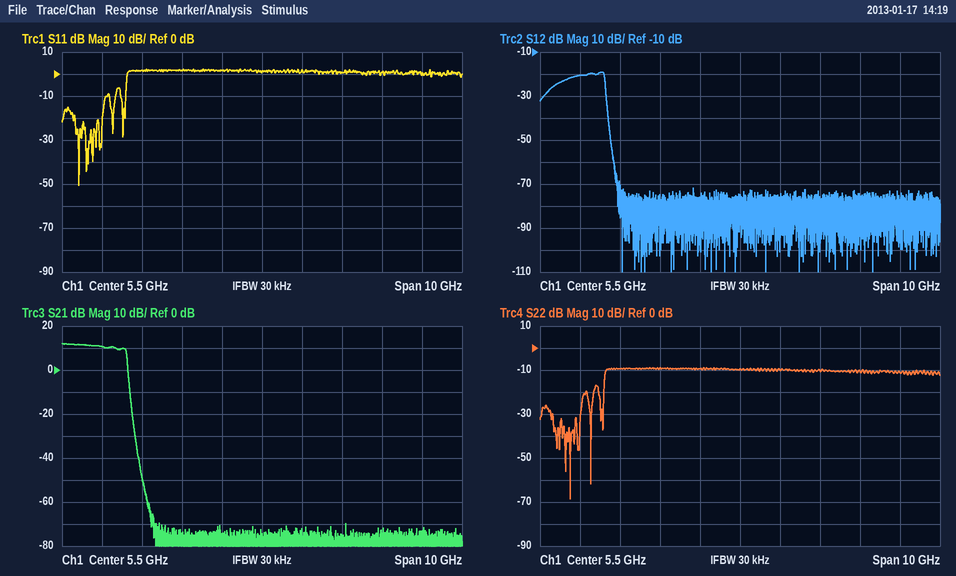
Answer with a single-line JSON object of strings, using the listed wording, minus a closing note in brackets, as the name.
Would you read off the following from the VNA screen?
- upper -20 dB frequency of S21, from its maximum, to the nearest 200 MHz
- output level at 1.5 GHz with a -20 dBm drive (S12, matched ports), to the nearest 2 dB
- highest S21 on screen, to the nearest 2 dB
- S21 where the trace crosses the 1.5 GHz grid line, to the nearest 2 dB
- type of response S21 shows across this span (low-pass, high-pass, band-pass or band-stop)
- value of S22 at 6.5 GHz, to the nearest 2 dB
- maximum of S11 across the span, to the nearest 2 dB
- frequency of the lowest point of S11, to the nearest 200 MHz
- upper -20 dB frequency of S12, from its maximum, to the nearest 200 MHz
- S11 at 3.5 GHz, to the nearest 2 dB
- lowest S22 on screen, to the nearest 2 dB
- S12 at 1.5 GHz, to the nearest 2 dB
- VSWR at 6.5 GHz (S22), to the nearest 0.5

{"upper -20 dB frequency of S21, from its maximum, to the nearest 200 MHz": "2.2 GHz", "output level at 1.5 GHz with a -20 dBm drive (S12, matched ports), to the nearest 2 dB": "-40 dBm", "highest S21 on screen, to the nearest 2 dB": "12 dB", "S21 where the trace crosses the 1.5 GHz grid line, to the nearest 2 dB": "10 dB", "type of response S21 shows across this span": "low-pass", "value of S22 at 6.5 GHz, to the nearest 2 dB": "-10 dB", "maximum of S11 across the span, to the nearest 2 dB": "2 dB", "frequency of the lowest point of S11, to the nearest 200 MHz": "1.0 GHz", "upper -20 dB frequency of S12, from its maximum, to the nearest 200 MHz": "2.2 GHz", "S11 at 3.5 GHz, to the nearest 2 dB": "2 dB", "lowest S22 on screen, to the nearest 2 dB": "-68 dB", "S12 at 1.5 GHz, to the nearest 2 dB": "-20 dB", "VSWR at 6.5 GHz (S22), to the nearest 0.5": "2.0"}
